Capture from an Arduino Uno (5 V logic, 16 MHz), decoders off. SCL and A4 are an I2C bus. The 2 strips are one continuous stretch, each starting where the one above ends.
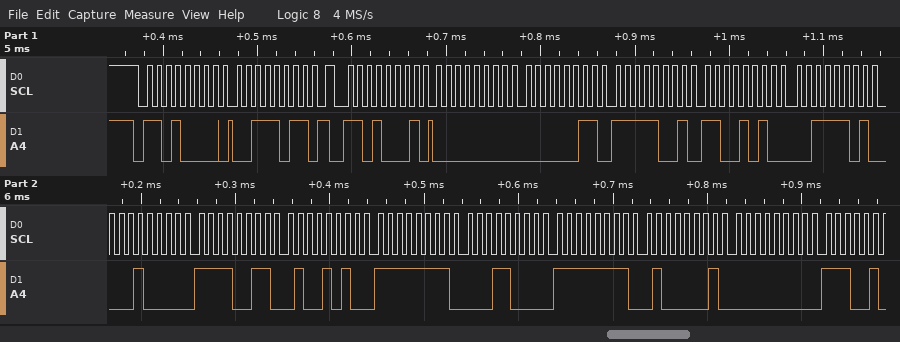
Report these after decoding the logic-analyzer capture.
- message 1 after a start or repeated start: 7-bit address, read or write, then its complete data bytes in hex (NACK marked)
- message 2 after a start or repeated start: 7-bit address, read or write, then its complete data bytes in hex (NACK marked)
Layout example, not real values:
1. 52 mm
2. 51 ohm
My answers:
1. 0x68 write: 3B
2. 0x68 read: 00 03 F9 CA 3D 10 F3 4A FF 18 FF 41 00
